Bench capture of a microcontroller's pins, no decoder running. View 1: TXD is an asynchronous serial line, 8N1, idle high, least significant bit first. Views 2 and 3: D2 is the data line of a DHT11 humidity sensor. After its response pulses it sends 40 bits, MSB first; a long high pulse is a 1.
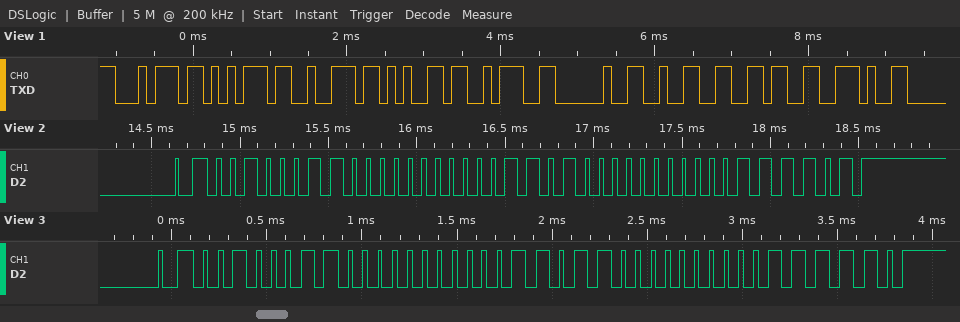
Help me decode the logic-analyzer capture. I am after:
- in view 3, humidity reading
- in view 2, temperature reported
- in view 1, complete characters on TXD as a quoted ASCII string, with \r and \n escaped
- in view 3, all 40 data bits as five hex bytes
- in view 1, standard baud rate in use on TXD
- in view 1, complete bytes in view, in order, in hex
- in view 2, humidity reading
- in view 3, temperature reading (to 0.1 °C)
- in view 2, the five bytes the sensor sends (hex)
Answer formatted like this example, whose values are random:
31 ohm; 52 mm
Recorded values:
35 %; 26.0 °C; "ture: 26."; 23 00 1B 00 3E; 9600 baud; 74 75 72 65 3A 20 32 36 2E; 35 %; 27.0 °C; 23 00 1A 00 3D
